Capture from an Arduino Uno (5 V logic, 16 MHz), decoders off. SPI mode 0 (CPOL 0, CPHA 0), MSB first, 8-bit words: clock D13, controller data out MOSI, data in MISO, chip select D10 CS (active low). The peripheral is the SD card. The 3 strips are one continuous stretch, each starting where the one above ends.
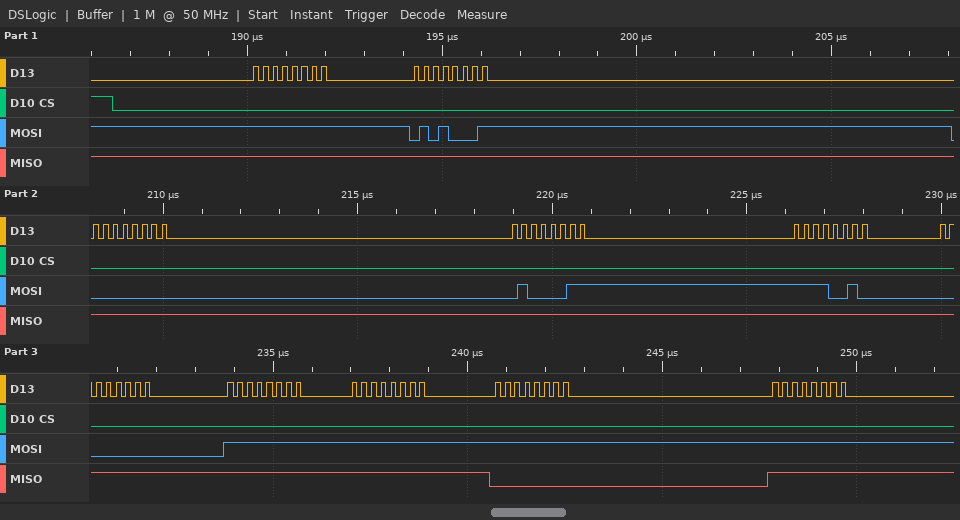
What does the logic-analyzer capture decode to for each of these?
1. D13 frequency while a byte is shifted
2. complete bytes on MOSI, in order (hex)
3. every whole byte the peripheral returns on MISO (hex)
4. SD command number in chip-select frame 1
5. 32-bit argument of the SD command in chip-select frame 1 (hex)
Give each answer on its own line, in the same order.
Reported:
4 MHz
0xFF 0x51 0x00 0x43 0xF2 0x00 0xFF 0xFF 0xFF 0xFF
0xFF 0xFF 0xFF 0xFF 0xFF 0xFF 0xFF 0xFF 0x00 0xFF
CMD17
0x0043F200
